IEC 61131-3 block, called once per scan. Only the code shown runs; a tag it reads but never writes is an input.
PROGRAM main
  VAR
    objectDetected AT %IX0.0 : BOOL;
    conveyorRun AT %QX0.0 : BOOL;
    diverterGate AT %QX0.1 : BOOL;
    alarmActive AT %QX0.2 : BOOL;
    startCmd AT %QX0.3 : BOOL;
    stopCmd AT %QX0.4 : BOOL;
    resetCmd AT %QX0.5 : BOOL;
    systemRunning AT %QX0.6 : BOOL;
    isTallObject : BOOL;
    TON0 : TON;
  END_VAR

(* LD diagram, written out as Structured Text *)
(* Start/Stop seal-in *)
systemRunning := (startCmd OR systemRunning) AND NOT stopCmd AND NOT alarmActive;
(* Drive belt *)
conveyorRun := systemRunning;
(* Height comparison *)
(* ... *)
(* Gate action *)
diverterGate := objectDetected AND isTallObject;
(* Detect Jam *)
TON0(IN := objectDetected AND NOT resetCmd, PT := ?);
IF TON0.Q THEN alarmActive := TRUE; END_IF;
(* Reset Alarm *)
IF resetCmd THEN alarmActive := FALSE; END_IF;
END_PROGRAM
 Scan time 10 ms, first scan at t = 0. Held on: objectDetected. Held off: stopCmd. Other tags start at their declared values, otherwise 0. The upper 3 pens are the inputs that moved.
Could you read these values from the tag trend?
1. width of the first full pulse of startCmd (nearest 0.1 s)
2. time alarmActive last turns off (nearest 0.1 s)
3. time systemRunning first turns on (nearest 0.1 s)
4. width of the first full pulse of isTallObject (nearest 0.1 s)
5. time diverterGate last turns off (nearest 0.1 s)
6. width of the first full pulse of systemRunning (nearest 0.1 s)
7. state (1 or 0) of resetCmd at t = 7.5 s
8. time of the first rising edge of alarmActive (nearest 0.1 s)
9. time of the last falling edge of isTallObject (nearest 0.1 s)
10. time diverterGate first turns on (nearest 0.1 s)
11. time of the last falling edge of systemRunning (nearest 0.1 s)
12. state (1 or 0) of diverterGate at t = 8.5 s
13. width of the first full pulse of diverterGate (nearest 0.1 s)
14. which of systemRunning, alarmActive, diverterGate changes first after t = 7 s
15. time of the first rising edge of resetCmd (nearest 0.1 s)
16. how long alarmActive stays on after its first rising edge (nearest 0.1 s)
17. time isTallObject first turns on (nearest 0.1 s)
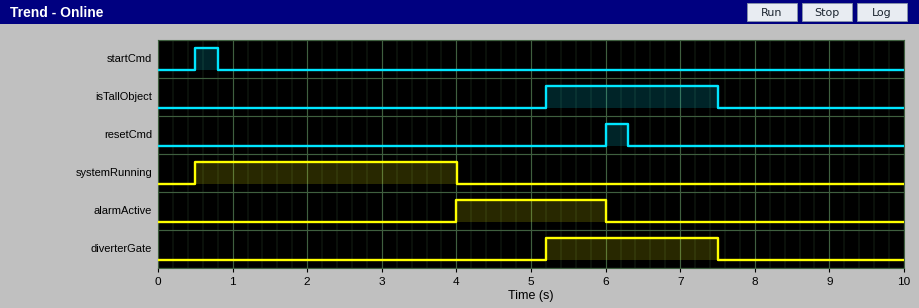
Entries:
0.3 s
6.0 s
0.5 s
2.3 s
7.5 s
3.5 s
0
4.0 s
7.5 s
5.2 s
4.0 s
0
2.3 s
diverterGate
6.0 s
2.0 s
5.2 s
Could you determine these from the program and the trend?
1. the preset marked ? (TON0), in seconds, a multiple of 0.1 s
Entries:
4.0 s
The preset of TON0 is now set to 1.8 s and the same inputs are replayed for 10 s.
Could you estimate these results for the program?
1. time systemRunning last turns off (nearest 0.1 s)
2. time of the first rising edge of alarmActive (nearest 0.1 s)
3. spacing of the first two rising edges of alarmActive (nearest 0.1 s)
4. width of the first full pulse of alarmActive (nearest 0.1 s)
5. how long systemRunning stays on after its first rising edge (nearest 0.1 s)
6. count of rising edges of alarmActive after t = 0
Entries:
1.8 s
1.8 s
6.3 s
4.2 s
1.3 s
2
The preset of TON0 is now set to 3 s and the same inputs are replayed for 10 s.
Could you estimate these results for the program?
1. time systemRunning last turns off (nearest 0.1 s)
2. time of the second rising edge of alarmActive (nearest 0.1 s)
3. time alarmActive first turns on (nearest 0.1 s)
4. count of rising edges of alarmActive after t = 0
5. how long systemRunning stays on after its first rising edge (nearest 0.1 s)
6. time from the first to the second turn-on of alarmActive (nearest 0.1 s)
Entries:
3.0 s
9.3 s
3.0 s
2
2.5 s
6.3 s
